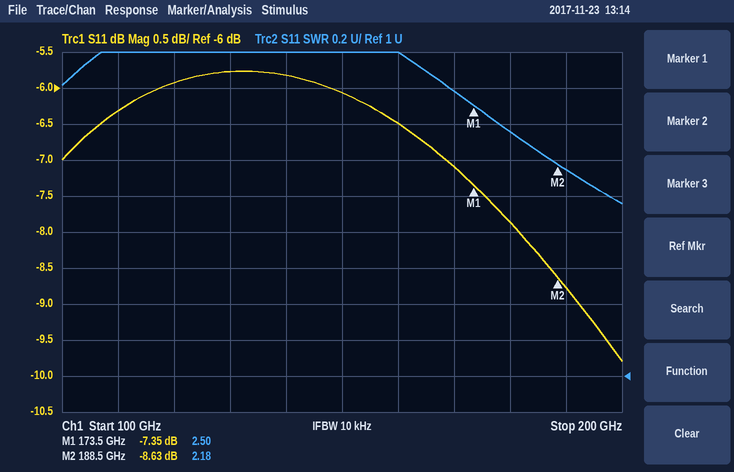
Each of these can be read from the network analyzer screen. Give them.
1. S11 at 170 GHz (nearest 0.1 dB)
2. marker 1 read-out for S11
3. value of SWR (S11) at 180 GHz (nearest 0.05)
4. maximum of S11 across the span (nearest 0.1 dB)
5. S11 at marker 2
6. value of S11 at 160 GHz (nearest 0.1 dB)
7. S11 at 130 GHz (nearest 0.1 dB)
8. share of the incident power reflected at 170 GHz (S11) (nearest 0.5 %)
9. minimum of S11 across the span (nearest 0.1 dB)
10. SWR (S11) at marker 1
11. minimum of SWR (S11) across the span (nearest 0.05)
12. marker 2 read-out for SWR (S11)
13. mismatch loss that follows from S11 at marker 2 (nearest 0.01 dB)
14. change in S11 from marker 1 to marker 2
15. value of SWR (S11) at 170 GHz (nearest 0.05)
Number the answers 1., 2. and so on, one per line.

1. -7.1 dB
2. -7.35 dB
3. 2.35
4. -5.8 dB
5. -8.63 dB
6. -6.5 dB
7. -5.8 dB
8. 19.5 %
9. -9.8 dB
10. 2.50
11. 1.95
12. 2.18
13. 0.64 dB
14. -1.28 dB
15. 2.60
